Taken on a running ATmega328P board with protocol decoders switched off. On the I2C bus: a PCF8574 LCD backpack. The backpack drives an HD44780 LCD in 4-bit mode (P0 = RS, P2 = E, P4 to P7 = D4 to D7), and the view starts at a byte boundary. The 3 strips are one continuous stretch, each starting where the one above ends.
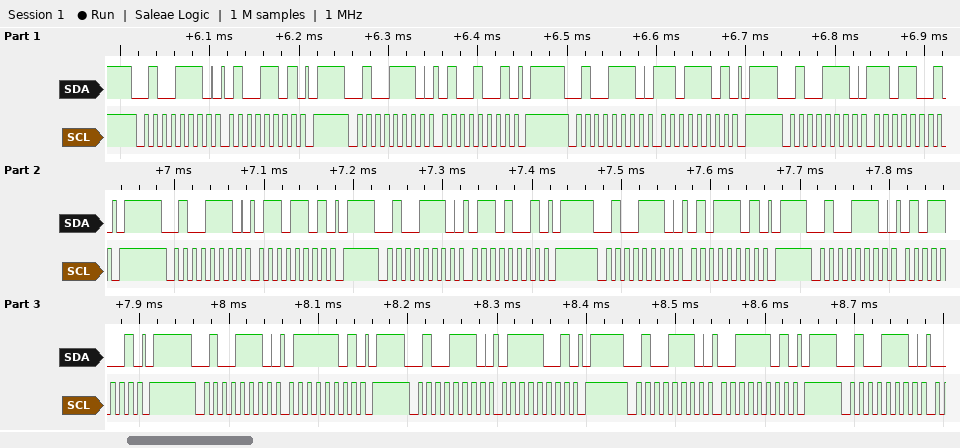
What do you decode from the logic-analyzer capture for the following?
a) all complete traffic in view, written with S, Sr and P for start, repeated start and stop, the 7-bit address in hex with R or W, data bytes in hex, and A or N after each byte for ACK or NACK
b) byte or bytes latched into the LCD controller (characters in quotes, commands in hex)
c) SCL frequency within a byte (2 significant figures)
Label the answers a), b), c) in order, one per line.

a) S 27W A 4D A P S 27W A 49 A P S 27W A DD A P S 27W A D9 A P S 27W A 6D A P S 27W A 69 A P S 27W A 5D A P S 27W A 59 A P S 27W A 7D A P S 27W A 79 A P S 27W A 3D A P S 27W A
b) 'M' 'e'
c) 100 kHz
